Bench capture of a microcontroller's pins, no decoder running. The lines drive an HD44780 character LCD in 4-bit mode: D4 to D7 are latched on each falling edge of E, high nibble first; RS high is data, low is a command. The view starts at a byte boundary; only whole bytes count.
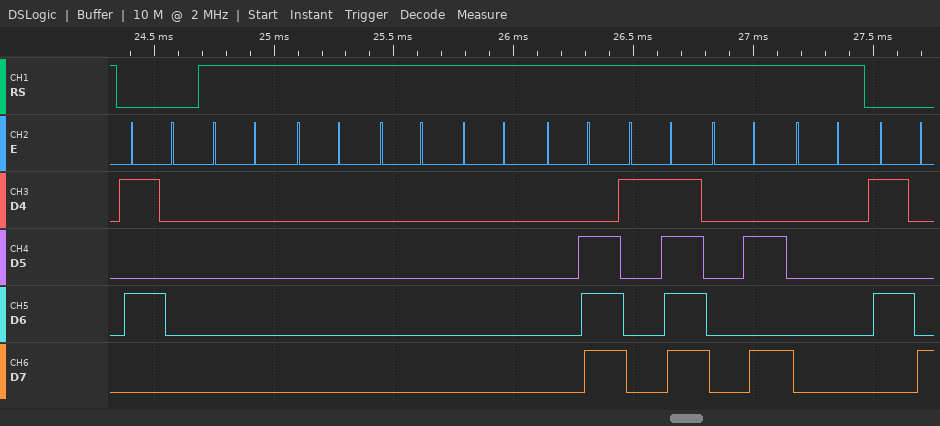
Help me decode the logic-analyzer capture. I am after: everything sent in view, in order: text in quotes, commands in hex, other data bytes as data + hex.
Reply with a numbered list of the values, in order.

1. 0x50 data 00 00 00 00 0E 1F 0A 00 0x58
